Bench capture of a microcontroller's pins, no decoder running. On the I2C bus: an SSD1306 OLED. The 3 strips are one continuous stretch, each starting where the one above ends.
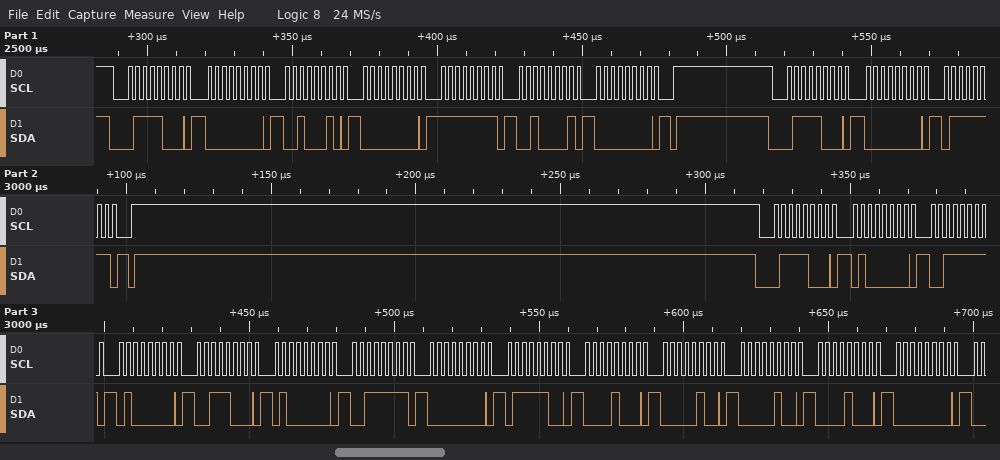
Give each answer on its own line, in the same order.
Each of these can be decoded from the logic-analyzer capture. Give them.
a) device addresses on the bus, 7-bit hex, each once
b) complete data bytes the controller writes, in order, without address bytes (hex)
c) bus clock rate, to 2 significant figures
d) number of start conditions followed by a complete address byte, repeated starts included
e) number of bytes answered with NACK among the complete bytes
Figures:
0x3C
00 22 00 FF 21 00 00 7F 40 3F 40 38 40 3F 00 7C 08 04 04 08 00
400 kHz
3
0
